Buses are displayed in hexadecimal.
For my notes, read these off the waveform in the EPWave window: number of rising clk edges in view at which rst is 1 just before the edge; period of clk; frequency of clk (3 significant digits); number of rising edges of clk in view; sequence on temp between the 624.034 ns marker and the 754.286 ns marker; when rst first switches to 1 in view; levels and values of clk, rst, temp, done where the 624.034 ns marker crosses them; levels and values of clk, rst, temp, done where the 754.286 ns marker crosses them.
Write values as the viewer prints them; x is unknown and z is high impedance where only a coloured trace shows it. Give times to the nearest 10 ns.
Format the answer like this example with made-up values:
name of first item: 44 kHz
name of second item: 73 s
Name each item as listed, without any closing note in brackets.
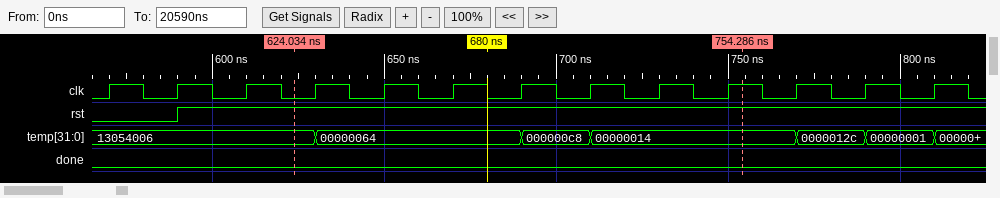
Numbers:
number of rising clk edges in view at which rst is 1 just before the edge: 11
period of clk: 20 ns
frequency of clk: 50.0 MHz
number of rising edges of clk in view: 13
sequence on temp between the 624.034 ns marker and the 754.286 ns marker: 13054006, 00000064, 000000c8, 00000014
when rst first switches to 1 in view: 590 ns
levels and values of clk, rst, temp, done where the 624.034 ns marker crosses them: clk=0, rst=1, temp=13054006, done=0
levels and values of clk, rst, temp, done where the 754.286 ns marker crosses them: clk=1, rst=1, temp=00000014, done=0
